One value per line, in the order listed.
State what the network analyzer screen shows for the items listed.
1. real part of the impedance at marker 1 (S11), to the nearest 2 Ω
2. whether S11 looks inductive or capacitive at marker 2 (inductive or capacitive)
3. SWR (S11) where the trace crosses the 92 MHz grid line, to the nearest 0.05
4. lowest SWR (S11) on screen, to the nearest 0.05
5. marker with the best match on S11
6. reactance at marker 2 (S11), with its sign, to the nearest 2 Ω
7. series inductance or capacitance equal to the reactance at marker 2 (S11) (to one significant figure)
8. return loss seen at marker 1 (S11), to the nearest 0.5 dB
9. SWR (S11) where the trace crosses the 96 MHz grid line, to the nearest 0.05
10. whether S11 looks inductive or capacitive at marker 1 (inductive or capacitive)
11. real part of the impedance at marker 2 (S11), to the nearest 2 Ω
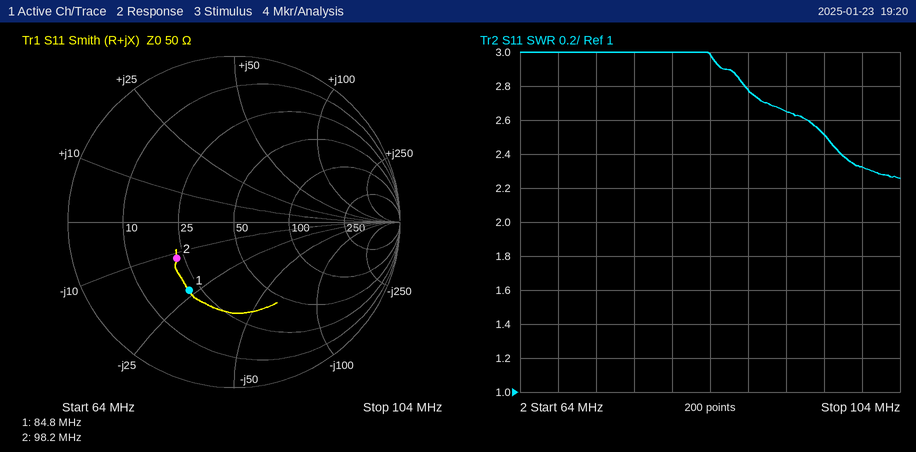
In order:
22 Ω
capacitive
2.65
2.25
marker 2
-12 Ω
100 pF
6.0 dB
2.50
capacitive
22 Ω
